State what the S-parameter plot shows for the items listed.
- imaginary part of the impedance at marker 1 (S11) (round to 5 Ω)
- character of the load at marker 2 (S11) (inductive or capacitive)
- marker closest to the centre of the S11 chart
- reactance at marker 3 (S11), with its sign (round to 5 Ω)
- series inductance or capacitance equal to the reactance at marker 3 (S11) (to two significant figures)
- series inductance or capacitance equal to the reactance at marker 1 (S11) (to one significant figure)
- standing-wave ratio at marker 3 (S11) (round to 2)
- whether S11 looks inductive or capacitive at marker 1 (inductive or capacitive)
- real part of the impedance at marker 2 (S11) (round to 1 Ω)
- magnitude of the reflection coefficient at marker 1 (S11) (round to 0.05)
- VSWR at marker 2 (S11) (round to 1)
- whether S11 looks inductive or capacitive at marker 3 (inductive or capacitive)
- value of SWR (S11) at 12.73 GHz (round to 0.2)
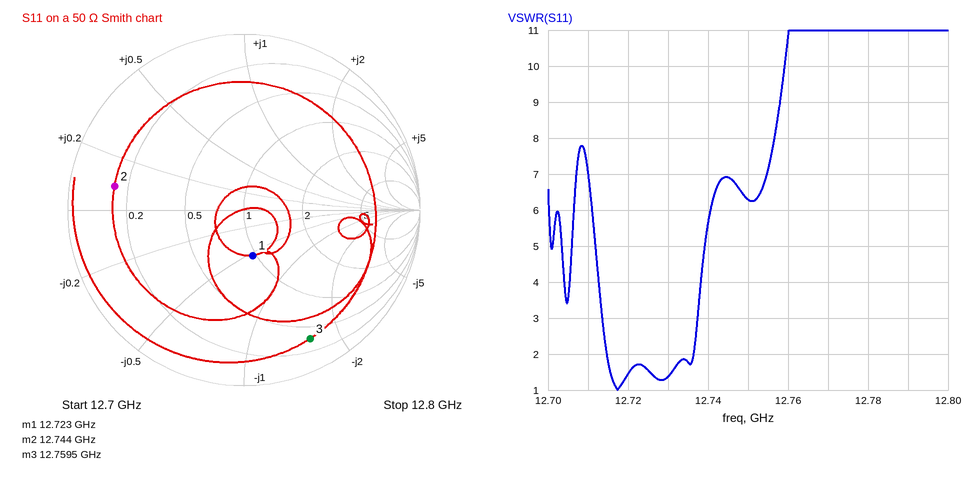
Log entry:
-25 Ω
inductive
marker 1
-80 Ω
160 fF
500 fF
10
capacitive
7 Ω
0.25
7
capacitive
1.4
